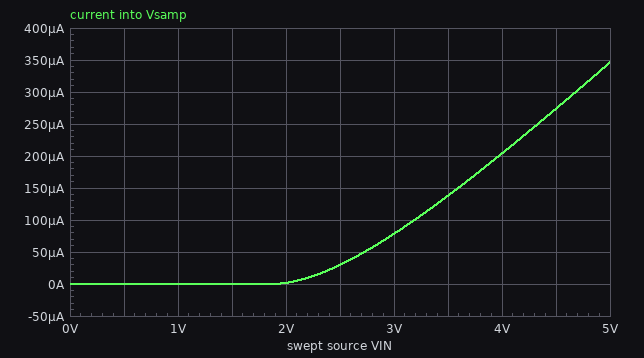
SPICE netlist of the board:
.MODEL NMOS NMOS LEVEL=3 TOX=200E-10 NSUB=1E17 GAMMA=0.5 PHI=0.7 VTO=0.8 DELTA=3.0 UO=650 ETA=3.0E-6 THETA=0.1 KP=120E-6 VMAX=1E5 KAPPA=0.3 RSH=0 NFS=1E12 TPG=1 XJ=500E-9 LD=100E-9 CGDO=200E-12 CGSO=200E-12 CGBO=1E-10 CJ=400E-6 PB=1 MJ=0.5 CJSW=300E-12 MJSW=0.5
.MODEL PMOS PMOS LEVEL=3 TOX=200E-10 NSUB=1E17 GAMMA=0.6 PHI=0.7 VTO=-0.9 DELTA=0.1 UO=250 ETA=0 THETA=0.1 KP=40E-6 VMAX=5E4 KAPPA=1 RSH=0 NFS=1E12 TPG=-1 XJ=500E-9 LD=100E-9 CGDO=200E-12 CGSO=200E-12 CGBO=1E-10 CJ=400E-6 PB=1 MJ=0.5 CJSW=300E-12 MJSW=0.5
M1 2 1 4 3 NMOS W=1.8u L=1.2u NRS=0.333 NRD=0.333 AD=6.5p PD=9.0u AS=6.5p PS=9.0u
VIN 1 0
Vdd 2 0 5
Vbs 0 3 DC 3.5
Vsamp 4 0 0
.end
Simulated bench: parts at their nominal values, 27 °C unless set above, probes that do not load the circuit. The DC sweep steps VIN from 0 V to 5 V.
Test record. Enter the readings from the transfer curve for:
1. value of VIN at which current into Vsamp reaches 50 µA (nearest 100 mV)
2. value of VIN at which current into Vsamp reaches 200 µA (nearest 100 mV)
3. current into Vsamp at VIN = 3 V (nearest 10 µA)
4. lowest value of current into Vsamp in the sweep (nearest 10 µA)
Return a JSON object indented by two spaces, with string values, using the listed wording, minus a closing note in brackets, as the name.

{
  "value of VIN at which current into Vsamp reaches 50 µA": "2.7 V",
  "value of VIN at which current into Vsamp reaches 200 µA": "4.0 V",
  "current into Vsamp at VIN = 3 V": "80 µA",
  "lowest value of current into Vsamp in the sweep": "0 A"
}
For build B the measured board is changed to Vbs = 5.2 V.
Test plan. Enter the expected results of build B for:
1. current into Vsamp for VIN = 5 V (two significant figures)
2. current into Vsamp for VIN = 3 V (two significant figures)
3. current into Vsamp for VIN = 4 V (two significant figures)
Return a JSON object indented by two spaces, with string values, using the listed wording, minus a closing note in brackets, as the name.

{
  "current into Vsamp for VIN = 5 V": "290 µA",
  "current into Vsamp for VIN = 3 V": "40 µA",
  "current into Vsamp for VIN = 4 V": "150 µA"
}
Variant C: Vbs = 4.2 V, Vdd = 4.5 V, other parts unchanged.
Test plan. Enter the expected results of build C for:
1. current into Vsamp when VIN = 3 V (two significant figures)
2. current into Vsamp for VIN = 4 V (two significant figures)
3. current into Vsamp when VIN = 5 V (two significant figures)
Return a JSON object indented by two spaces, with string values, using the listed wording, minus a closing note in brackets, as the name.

{
  "current into Vsamp when VIN = 3 V": "61 µA",
  "current into Vsamp for VIN = 4 V": "180 µA",
  "current into Vsamp when VIN = 5 V": "320 µA"
}
